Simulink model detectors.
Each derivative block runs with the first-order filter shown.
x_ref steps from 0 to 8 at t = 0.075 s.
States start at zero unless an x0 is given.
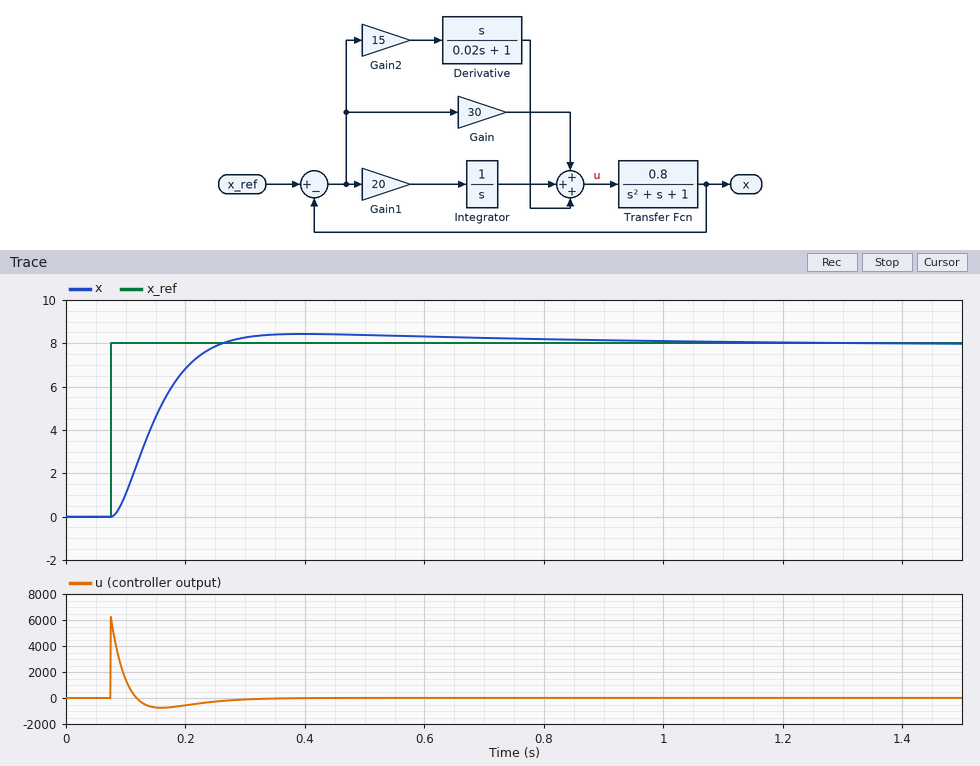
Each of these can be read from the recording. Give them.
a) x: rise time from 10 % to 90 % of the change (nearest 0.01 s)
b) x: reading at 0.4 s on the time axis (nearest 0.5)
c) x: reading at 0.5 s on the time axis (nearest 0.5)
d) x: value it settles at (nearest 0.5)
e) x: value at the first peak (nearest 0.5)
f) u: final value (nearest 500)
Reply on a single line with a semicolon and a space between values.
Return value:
0.12 s; 8.5; 8.5; 8.0; 8.5; 0
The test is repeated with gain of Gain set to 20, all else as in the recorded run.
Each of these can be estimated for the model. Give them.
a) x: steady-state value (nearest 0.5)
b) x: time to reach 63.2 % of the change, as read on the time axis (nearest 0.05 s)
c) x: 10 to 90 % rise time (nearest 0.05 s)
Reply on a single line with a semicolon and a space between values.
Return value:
8.0; 0.15 s; 0.15 s
